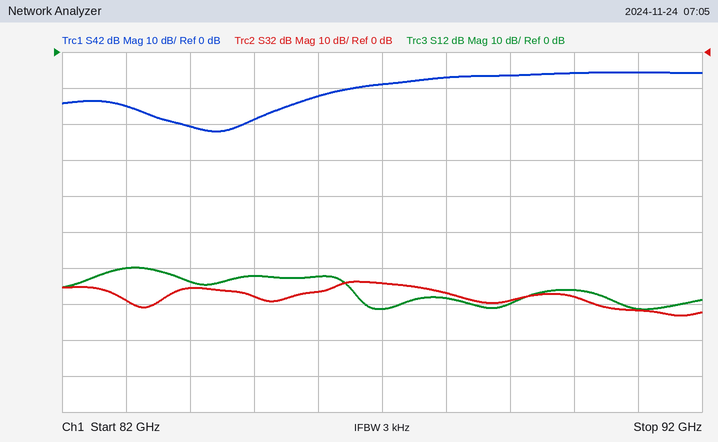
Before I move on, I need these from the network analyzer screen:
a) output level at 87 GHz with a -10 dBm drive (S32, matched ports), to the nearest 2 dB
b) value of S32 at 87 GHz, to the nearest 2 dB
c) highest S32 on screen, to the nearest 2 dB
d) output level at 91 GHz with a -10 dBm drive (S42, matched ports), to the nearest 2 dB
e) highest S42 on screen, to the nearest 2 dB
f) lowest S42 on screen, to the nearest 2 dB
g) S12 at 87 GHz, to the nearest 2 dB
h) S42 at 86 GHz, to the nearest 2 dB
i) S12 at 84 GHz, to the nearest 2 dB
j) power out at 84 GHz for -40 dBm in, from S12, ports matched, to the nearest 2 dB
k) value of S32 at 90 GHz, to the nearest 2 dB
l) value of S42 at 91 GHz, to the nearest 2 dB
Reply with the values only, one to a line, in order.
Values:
-74 dBm
-64 dB
-64 dB
-16 dBm
-6 dB
-22 dB
-72 dB
-12 dB
-64 dB
-104 dBm
-68 dB
-6 dB
